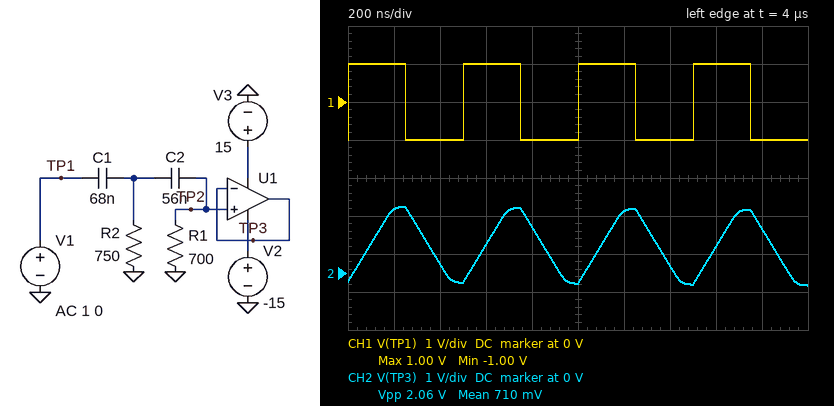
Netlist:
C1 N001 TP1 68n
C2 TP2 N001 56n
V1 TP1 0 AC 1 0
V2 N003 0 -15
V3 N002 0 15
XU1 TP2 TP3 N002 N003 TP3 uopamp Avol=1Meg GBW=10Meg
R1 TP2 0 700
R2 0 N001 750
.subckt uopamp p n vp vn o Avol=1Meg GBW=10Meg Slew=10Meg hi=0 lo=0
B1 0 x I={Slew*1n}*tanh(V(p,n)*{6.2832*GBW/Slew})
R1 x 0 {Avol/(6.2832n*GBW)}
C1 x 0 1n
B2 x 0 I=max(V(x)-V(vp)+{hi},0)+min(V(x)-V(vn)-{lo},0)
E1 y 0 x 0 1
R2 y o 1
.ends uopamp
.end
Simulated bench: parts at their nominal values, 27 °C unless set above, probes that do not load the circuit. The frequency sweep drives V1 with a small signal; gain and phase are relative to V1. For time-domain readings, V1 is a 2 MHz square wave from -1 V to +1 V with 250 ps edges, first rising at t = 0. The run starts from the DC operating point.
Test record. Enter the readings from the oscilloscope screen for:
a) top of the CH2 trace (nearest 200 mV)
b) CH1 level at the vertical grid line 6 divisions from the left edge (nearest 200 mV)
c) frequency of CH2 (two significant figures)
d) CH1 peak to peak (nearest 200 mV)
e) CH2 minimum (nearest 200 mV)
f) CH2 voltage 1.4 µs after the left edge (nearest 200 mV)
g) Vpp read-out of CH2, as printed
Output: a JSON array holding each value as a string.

["1.8 V", "1.0 V", "2.0 MHz", "2.0 V", "-400 mV", "200 mV", "2.06 V"]
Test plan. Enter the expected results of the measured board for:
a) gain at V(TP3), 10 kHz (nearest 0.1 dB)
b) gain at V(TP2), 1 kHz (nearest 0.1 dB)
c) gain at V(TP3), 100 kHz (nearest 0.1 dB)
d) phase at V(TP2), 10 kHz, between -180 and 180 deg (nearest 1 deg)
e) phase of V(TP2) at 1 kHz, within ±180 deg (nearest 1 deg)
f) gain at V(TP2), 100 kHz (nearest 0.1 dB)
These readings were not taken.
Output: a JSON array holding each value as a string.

["-2.7 dB", "-23.9 dB", "0 dB", "50 deg", "138 deg", "0 dB"]
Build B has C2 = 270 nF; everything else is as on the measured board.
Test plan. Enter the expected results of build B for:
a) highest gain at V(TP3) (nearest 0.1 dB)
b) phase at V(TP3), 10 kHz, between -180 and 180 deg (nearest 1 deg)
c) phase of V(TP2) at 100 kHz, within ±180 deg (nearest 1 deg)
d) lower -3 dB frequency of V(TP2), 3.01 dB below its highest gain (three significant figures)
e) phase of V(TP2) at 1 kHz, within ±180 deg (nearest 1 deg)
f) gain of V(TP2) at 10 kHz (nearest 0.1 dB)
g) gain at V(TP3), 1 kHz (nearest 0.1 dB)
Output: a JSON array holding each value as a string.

["0 dB", "37 deg", "4 deg", "6.95 kHz", "103 deg", "-1.7 dB", "-17.5 dB"]
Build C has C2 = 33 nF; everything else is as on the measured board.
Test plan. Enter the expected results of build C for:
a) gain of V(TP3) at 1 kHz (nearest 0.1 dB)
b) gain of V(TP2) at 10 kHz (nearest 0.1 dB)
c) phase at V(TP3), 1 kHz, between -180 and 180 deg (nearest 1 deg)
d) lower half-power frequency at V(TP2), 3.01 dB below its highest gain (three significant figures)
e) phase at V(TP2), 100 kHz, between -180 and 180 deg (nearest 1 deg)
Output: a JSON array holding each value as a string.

["-27.8 dB", "-3.8 dB", "147 deg", "11.8 kHz", "8 deg"]
